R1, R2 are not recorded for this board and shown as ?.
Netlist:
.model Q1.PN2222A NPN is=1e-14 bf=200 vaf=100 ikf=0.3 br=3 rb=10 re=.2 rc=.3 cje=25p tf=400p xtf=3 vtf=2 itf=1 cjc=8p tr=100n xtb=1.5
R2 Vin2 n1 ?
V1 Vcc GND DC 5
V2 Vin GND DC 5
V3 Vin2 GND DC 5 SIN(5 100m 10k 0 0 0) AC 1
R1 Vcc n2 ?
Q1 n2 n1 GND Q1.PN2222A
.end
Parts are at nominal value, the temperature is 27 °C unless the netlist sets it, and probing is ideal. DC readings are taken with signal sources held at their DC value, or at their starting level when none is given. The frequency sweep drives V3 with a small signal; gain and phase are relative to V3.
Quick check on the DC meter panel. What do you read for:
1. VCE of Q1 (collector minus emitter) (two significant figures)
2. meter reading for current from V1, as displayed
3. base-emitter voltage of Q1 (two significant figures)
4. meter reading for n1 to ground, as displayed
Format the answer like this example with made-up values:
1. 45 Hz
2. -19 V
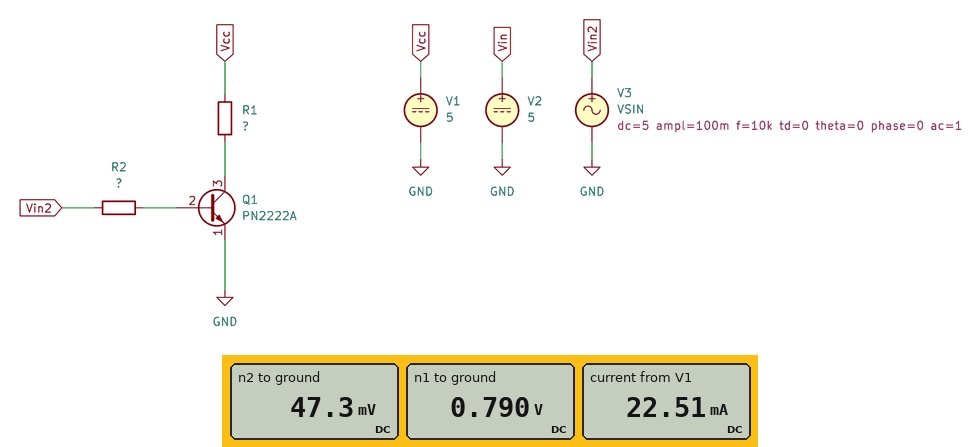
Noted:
1. 47 mV
2. 22.51 mA
3. 790 mV
4. 0.790 V
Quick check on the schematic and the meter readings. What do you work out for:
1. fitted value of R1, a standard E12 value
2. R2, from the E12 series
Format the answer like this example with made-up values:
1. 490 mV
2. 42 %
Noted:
1. 220 Ω
2. 1.2 kΩ
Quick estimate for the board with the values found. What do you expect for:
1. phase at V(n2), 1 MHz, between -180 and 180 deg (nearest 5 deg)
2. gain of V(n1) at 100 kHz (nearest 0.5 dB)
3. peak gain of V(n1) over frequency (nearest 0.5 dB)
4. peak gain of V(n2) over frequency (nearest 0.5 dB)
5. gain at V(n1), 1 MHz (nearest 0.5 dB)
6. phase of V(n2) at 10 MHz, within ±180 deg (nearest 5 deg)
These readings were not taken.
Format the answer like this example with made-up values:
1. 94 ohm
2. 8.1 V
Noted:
1. 95 deg
2. -39.5 dB
3. -39.5 dB
4. -48.5 dB
5. -40.5 dB
6. 15 deg
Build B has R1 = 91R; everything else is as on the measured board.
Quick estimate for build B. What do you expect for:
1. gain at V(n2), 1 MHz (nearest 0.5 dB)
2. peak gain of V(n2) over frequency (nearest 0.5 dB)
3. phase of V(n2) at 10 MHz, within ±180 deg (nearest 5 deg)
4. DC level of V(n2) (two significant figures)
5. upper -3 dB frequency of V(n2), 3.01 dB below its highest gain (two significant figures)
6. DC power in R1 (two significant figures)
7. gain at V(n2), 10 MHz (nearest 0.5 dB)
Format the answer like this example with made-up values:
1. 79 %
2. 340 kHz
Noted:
1. -52.0 dB
2. -45.5 dB
3. 30 deg
4. 83 mV
5. 540 kHz
6. 270 mW
7. -64.5 dB
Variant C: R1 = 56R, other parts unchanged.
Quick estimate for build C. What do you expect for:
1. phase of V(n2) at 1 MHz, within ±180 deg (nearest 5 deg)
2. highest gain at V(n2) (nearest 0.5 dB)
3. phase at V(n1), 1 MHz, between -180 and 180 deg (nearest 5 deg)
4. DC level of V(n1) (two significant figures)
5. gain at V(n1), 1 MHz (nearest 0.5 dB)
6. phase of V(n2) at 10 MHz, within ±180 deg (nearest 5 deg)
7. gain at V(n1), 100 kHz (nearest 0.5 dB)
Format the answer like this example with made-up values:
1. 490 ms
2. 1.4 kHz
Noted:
1. 110 deg
2. -44.0 dB
3. 0 deg
4. 830 mV
5. -41.0 dB
6. 40 deg
7. -40.5 dB
